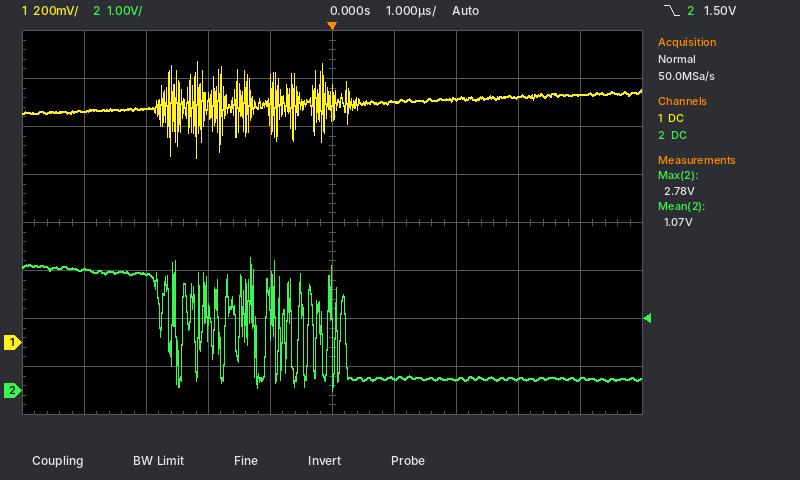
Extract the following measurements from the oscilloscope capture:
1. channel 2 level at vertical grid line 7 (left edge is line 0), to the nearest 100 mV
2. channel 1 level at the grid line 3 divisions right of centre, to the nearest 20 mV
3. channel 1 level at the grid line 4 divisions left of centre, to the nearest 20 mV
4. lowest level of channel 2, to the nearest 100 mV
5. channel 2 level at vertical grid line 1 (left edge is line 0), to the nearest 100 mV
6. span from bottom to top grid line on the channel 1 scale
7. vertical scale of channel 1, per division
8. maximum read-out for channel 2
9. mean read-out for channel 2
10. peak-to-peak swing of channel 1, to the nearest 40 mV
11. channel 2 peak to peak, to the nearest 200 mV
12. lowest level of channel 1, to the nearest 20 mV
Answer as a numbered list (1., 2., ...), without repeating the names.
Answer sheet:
1. 200 mV
2. 1.02 V
3. 960 mV
4. 0.0 V
5. 2.5 V
6. 1.6 V
7. 200 mV
8. 2.78 V
9. 1.07 V
10. 400 mV
11. 2.8 V
12. 780 mV
